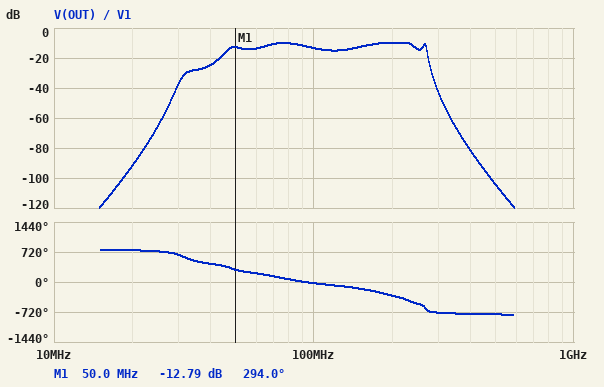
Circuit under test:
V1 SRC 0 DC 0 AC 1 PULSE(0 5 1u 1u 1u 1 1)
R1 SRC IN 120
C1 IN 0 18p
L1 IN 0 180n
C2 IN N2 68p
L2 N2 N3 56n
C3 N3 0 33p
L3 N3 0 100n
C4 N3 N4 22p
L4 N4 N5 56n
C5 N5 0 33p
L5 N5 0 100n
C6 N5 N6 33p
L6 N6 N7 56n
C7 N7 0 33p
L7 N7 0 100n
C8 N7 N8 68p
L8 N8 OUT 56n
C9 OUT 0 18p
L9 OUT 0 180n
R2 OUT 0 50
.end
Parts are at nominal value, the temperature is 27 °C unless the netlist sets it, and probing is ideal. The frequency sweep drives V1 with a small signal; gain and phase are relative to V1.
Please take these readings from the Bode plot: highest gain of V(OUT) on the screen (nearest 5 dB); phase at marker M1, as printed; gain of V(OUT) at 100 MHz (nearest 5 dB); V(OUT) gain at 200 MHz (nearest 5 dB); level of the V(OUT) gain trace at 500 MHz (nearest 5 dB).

-10 dB
294.0 deg
-15 dB
-10 dB
-105 dB
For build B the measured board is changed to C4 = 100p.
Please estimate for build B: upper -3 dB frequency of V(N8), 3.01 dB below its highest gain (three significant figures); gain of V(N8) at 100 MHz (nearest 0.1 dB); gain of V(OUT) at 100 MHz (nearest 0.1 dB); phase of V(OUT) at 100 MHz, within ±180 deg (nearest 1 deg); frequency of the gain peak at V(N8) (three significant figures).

260 MHz
-10.1 dB
-11.4 dB
-47 deg
255 MHz
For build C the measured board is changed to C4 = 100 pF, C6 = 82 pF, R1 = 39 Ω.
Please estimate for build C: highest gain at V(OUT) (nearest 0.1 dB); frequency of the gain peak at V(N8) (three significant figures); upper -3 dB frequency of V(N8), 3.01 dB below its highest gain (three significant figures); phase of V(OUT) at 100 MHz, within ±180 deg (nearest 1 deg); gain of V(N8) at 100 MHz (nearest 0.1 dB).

-5.0 dB
244 MHz
251 MHz
-62 deg
-3.9 dB
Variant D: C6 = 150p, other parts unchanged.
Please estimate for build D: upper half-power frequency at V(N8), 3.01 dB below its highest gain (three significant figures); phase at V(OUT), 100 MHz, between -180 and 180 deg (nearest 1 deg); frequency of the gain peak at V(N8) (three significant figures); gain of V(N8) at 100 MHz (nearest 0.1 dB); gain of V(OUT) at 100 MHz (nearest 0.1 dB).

267 MHz
-44 deg
263 MHz
-10.3 dB
-11.5 dB
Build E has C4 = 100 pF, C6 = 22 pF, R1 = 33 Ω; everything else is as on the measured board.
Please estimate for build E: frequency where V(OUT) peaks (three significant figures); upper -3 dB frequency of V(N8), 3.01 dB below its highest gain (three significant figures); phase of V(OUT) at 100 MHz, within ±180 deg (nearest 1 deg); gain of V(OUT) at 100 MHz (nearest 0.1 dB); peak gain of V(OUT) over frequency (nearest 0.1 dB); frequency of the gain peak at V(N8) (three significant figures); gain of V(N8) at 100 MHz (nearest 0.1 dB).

107 MHz
264 MHz
-30 deg
-4.6 dB
-4.5 dB
260 MHz
-3.3 dB
